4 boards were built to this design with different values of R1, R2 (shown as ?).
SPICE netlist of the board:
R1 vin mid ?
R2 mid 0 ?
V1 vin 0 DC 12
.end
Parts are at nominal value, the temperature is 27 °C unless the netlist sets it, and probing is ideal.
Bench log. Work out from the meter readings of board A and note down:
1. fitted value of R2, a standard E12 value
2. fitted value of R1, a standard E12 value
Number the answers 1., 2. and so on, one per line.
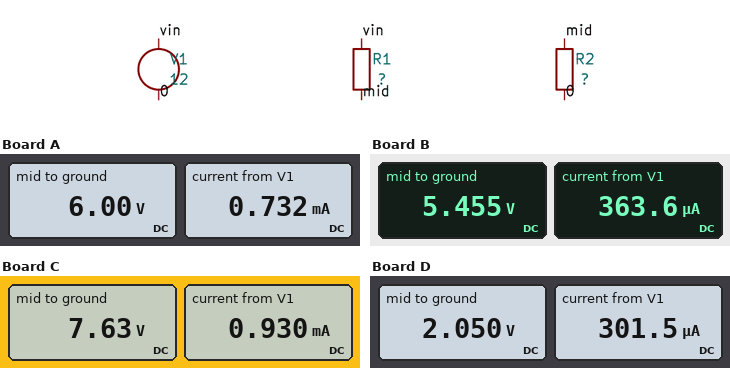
1. 8.2 kΩ
2. 8.2 kΩ
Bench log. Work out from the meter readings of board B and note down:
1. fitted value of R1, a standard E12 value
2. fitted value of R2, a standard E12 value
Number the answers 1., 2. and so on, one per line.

1. 18 kΩ
2. 15 kΩ
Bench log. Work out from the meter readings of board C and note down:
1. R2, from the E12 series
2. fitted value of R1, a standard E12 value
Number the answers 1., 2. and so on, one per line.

1. 8.2 kΩ
2. 4.7 kΩ
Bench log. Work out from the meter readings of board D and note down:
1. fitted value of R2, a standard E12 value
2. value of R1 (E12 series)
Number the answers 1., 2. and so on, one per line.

1. 6.8 kΩ
2. 33 kΩ
